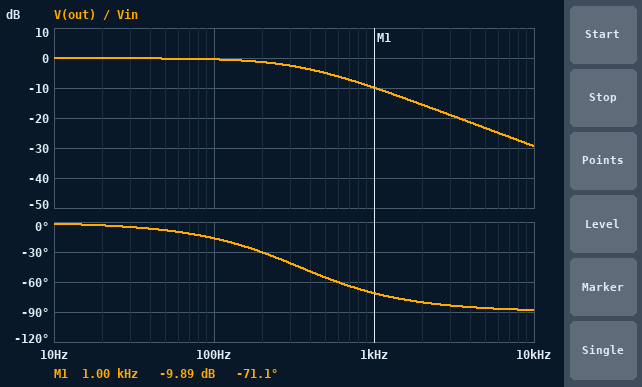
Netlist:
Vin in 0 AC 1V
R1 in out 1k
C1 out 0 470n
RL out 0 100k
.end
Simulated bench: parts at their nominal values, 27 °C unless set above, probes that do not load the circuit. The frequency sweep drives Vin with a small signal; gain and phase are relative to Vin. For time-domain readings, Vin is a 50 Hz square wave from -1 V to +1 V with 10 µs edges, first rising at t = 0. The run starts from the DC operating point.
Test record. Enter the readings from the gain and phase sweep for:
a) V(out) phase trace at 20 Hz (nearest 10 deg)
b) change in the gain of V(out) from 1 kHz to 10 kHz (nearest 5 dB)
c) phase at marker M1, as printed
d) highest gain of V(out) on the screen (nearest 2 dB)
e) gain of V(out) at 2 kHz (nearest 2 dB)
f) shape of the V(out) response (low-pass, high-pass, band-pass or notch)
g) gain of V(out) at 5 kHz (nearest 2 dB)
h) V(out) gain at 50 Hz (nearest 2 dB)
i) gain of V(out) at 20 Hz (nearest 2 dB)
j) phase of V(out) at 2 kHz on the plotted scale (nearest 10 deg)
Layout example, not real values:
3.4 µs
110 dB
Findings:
0 deg
-20 dB
-71.1 deg
0 dB
-16 dB
low-pass
-24 dB
0 dB
0 dB
-80 deg
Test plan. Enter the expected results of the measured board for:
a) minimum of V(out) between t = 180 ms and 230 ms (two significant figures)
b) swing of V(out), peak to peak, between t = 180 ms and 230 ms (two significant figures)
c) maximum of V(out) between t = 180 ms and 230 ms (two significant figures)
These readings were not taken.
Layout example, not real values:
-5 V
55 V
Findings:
-990 mV
2.0 V
990 mV
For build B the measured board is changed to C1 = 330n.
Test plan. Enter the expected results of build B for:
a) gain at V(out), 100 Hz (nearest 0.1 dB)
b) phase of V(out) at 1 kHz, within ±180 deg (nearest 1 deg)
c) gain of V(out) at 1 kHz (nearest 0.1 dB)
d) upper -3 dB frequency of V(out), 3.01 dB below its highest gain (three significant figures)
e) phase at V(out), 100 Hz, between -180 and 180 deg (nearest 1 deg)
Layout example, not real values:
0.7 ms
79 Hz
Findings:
-0.3 dB
-64 deg
-7.3 dB
487 Hz
-12 deg
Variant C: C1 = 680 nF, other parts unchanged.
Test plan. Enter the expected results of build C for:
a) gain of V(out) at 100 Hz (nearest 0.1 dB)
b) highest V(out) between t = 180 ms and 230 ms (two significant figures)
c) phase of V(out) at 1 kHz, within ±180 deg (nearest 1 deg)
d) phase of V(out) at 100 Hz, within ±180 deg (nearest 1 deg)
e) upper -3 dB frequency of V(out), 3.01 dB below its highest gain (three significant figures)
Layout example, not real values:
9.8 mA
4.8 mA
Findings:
-0.8 dB
990 mV
-77 deg
-23 deg
236 Hz
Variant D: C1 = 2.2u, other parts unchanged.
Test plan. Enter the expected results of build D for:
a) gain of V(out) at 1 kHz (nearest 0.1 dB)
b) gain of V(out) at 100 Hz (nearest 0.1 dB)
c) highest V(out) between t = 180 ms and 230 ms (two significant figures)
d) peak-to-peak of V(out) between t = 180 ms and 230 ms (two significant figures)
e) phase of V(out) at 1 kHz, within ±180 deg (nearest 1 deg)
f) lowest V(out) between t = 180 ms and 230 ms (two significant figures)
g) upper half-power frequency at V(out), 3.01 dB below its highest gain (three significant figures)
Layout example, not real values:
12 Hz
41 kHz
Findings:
-22.8 dB
-4.7 dB
970 mV
1.9 V
-86 deg
-970 mV
73.1 Hz
